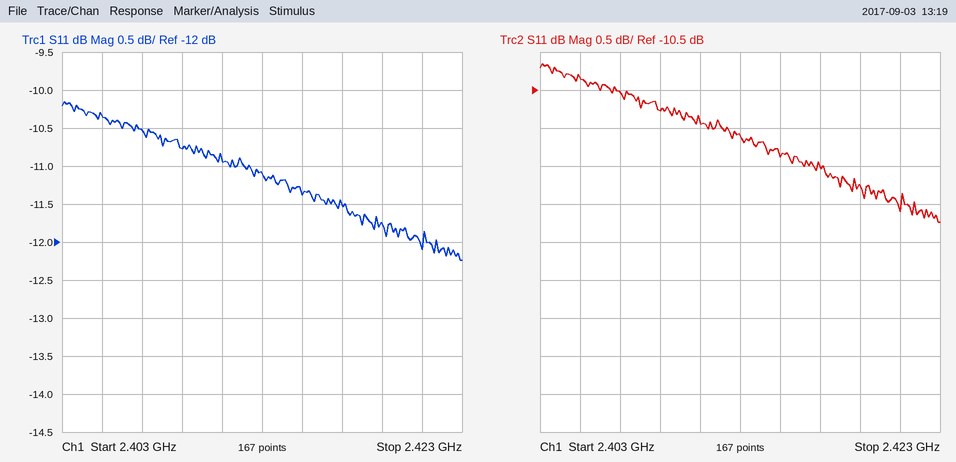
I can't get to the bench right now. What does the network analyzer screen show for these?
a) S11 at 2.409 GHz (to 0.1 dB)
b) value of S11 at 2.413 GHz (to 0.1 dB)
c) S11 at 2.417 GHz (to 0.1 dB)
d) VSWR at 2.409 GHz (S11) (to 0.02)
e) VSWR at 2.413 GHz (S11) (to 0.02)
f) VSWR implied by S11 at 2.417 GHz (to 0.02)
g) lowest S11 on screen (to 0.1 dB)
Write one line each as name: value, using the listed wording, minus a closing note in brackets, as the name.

S11 at 2.409 GHz: -10.8 dB
value of S11 at 2.413 GHz: -11.1 dB
S11 at 2.417 GHz: -11.5 dB
VSWR at 2.409 GHz (S11): 1.82
VSWR at 2.413 GHz (S11): 1.78
VSWR implied by S11 at 2.417 GHz: 1.72
lowest S11 on screen: -12.2 dB
